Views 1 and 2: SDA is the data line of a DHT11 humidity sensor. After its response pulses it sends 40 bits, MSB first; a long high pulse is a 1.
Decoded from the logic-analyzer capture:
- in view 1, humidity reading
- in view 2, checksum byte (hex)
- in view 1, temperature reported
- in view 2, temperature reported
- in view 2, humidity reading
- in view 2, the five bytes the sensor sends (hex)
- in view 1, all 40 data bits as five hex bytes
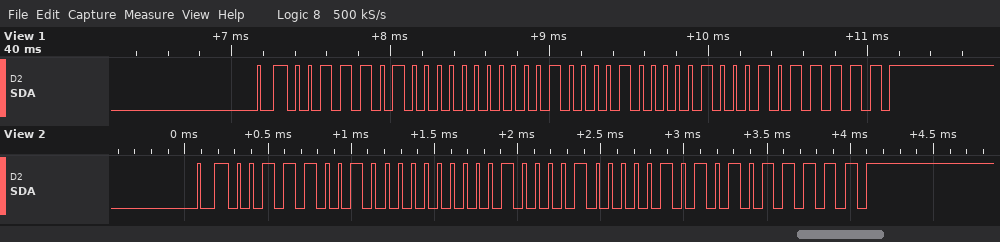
58 %
0x5F
33.4 °C
33.5 °C
57 %
39 00 21 05 5F
3A 00 21 04 5F
